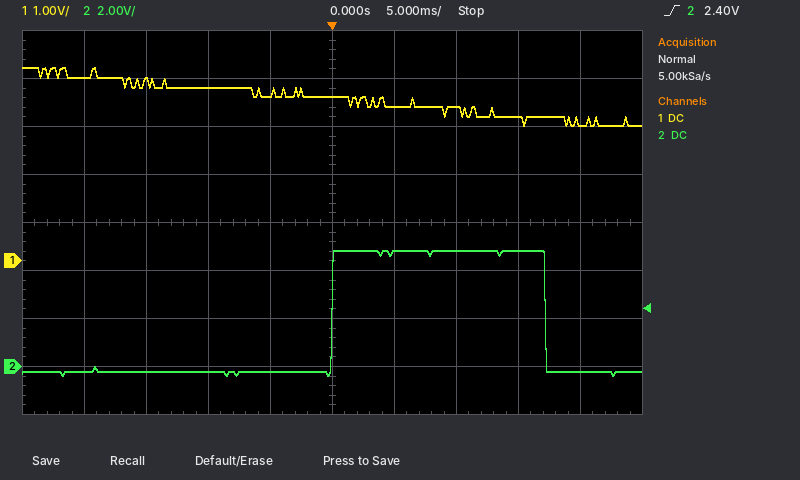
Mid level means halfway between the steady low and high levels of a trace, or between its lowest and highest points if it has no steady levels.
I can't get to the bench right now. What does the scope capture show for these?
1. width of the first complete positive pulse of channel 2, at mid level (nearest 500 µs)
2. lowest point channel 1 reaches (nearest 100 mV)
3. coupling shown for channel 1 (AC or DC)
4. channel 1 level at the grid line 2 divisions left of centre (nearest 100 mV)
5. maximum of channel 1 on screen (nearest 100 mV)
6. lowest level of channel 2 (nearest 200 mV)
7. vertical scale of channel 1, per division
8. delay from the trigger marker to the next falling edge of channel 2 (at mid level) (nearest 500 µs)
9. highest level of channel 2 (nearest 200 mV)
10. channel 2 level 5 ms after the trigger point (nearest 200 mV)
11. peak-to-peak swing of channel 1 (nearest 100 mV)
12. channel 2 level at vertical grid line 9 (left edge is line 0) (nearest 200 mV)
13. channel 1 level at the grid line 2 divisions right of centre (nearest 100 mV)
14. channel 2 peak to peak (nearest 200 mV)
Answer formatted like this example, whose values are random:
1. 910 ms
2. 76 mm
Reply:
1. 17.0 ms
2. 2.8 V
3. DC
4. 3.6 V
5. 4.0 V
6. -400 mV
7. 1 V
8. 17.0 ms
9. 4.8 V
10. 4.8 V
11. 1.2 V
12. -200 mV
13. 3.2 V
14. 5.2 V
